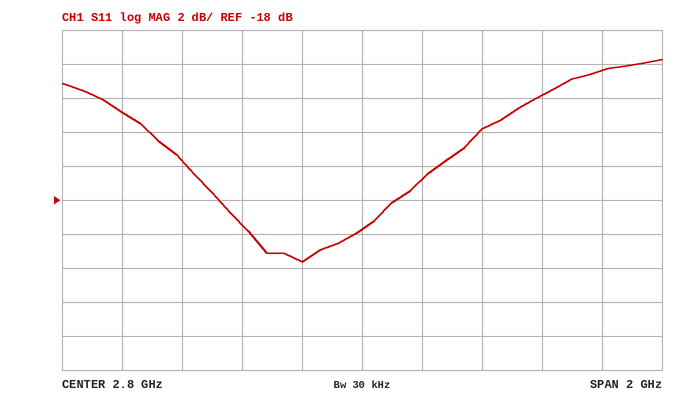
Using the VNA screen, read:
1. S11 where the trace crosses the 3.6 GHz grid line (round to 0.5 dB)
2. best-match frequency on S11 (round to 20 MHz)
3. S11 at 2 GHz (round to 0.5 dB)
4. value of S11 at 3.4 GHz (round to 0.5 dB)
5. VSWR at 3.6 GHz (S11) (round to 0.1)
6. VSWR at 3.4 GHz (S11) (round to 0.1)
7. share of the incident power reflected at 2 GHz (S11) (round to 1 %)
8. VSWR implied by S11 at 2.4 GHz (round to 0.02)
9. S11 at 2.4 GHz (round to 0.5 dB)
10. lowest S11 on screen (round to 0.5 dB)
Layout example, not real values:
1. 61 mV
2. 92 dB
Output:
1. -10.5 dB
2. 2.60 GHz
3. -13.0 dB
4. -12.0 dB
5. 1.9
6. 1.7
7. 5 %
8. 1.24
9. -19.5 dB
10. -21.5 dB
